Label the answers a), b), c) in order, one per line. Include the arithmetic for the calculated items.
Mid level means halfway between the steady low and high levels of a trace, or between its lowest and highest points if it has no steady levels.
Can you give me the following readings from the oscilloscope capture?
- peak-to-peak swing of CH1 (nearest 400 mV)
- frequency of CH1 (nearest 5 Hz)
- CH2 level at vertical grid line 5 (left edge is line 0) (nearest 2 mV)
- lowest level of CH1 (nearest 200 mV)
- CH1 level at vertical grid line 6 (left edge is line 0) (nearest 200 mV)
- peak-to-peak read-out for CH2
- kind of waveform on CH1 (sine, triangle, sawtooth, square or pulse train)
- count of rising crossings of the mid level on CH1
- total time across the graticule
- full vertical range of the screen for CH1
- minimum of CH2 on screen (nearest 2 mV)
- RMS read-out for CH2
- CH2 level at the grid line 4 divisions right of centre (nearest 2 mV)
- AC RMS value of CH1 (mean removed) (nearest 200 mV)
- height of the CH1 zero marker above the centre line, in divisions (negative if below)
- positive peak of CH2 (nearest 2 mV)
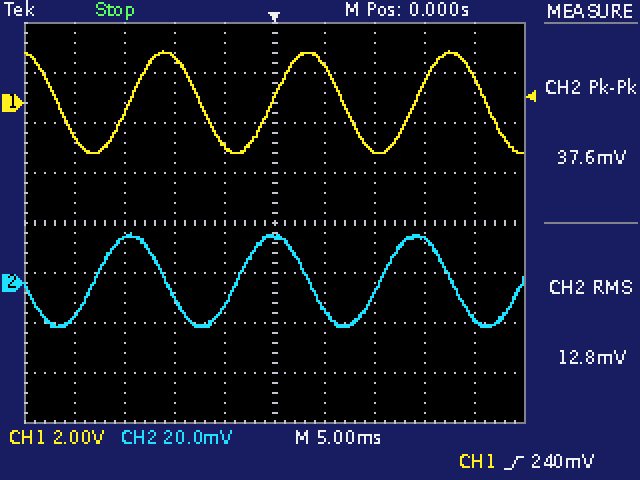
a) 4.0 V
b) 70 Hz
c) 18 mV
d) -2.0 V
e) 1.4 V
f) 37.6 mV
g) sine
h) 3
i) 50 ms
j) 16 V
k) -18 mV
l) 12.8 mV
m) -14 mV
n) 4.0 V / (2√2) ≈ 1.4 V
o) +2.4 div
p) 20 mV
